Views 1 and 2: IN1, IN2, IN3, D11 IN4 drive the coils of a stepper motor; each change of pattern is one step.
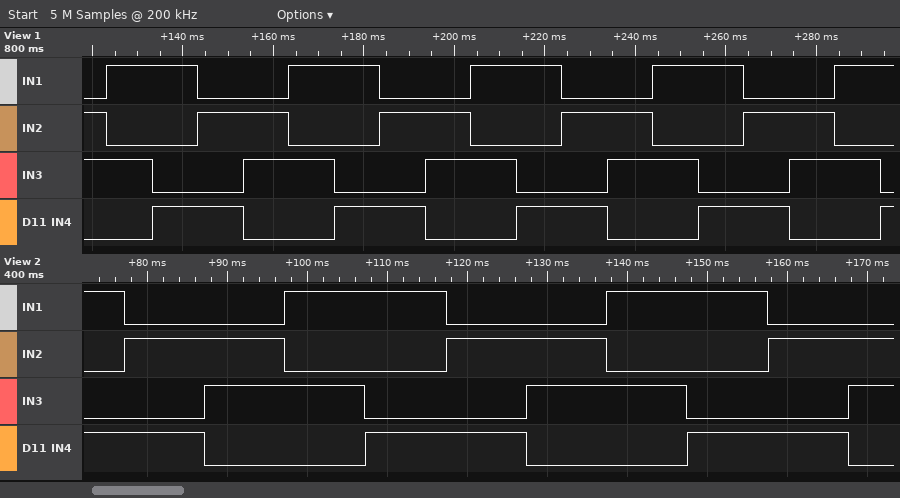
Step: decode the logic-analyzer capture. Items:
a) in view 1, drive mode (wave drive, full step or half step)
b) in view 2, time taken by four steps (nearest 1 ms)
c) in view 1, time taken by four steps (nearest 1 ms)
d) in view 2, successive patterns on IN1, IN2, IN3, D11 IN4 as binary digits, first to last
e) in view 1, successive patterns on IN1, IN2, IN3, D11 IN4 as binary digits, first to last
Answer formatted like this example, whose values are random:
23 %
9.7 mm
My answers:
full step
40 ms
40 ms
1001 0101 0110 1010 1001 0101 0110 1010 1001 0101 0110
0110 1010 1001 0101 0110 1010 1001 0101 0110 1010 1001 0101 0110 1010 1001 0101 0110 1010 1001
